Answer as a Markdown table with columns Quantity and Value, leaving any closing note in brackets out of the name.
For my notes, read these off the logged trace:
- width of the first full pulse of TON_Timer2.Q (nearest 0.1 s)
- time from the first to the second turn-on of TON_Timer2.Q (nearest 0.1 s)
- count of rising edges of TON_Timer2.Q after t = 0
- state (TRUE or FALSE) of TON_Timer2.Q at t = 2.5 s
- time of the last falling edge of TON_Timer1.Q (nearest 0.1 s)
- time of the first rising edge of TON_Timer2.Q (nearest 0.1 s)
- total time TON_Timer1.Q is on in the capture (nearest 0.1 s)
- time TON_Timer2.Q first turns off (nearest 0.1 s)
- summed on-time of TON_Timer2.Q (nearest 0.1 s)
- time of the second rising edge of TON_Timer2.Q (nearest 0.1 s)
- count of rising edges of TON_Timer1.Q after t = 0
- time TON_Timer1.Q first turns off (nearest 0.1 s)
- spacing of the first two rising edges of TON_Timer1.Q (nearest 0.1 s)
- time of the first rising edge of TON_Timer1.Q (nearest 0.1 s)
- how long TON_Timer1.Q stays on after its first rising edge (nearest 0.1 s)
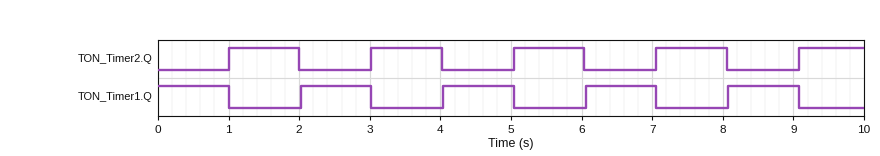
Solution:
| Quantity | Value |
|---|---|
| width of the first full pulse of TON_Timer2.Q | 1.0 s |
| time from the first to the second turn-on of TON_Timer2.Q | 2.0 s |
| count of rising edges of TON_Timer2.Q after t = 0 | 5 |
| state (TRUE or FALSE) of TON_Timer2.Q at t = 2.5 s | FALSE |
| time of the last falling edge of TON_Timer1.Q | 9.1 s |
| time of the first rising edge of TON_Timer2.Q | 1.0 s |
| total time TON_Timer1.Q is on in the capture | 5.0 s |
| time TON_Timer2.Q first turns off | 2.0 s |
| summed on-time of TON_Timer2.Q | 4.9 s |
| time of the second rising edge of TON_Timer2.Q | 3.0 s |
| count of rising edges of TON_Timer1.Q after t = 0 | 4 |
| time TON_Timer1.Q first turns off | 1.0 s |
| spacing of the first two rising edges of TON_Timer1.Q | 2.0 s |
| time of the first rising edge of TON_Timer1.Q | 2.0 s |
| how long TON_Timer1.Q stays on after its first rising edge | 1.0 s |
